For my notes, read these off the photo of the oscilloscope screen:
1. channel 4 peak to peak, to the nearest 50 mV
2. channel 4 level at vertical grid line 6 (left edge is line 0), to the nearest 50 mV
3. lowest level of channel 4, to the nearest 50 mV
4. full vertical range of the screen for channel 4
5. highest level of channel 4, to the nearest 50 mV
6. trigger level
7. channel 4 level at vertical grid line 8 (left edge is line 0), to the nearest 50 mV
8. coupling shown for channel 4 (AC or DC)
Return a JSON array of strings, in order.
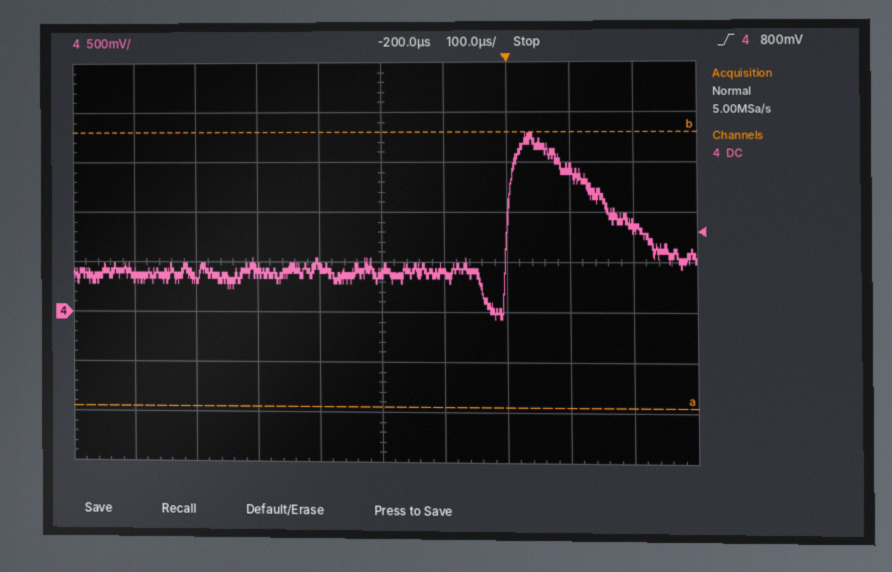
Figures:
["1.85 V", "400 mV", "-50 mV", "4 V", "1.80 V", "800 mV", "1.45 V", "DC"]
